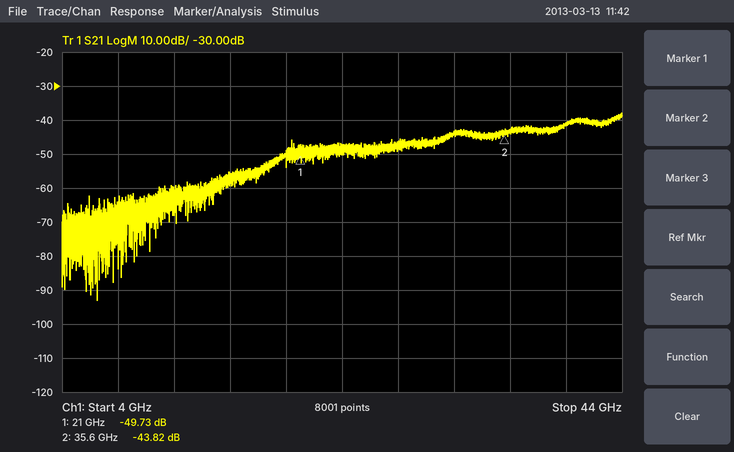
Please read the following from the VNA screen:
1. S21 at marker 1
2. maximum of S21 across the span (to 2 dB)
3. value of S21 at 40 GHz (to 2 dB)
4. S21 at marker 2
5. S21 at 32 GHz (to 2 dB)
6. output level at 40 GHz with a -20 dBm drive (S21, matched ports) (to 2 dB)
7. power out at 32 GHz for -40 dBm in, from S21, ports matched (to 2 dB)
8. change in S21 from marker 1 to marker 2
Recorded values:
-49.73 dB
-38 dB
-42 dB
-43.82 dB
-44 dB
-62 dBm
-84 dBm
5.91 dB
